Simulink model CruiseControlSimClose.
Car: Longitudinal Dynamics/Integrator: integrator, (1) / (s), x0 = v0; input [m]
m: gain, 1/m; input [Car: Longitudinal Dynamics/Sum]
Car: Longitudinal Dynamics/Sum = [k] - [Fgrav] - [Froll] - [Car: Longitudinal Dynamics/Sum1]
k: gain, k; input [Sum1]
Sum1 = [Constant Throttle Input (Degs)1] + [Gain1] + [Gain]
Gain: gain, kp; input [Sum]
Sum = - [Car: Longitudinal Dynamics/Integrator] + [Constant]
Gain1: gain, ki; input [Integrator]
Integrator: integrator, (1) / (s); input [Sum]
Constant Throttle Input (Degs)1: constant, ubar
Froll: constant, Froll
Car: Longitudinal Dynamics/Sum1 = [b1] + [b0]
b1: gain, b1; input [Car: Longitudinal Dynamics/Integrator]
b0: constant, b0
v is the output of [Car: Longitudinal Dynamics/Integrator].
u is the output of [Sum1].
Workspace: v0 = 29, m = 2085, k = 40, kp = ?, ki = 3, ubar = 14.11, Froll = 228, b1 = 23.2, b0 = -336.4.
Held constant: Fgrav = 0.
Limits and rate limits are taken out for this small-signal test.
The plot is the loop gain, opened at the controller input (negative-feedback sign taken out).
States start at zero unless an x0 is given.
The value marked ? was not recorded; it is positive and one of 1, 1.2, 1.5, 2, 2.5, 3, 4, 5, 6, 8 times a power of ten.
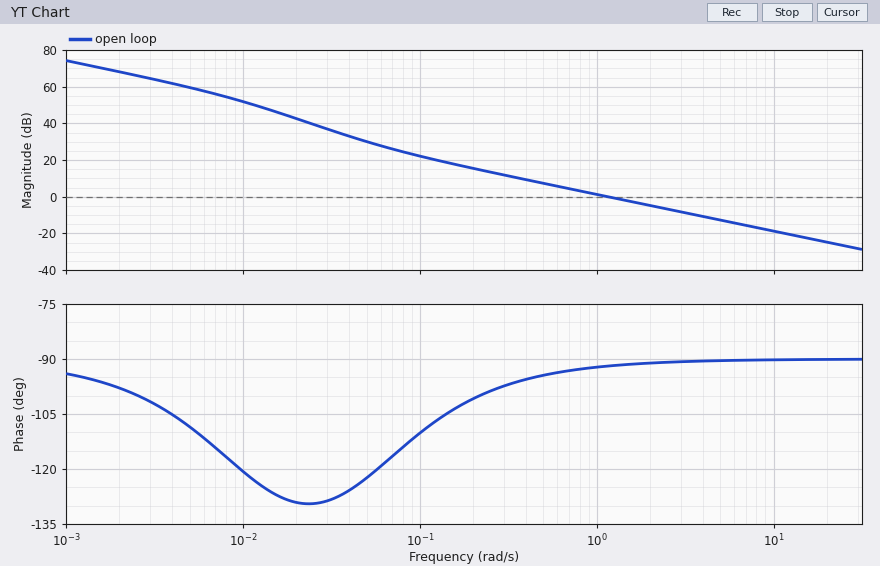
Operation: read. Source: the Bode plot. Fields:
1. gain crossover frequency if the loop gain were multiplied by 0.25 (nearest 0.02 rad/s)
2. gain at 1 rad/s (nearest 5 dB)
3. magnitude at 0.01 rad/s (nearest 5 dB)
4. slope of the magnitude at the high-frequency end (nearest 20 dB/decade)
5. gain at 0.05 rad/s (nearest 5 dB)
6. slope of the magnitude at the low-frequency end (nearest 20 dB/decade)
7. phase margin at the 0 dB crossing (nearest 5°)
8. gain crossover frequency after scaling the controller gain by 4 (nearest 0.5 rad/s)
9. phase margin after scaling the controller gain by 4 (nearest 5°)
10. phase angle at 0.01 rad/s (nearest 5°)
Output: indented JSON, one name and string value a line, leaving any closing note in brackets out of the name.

{
  "gain crossover frequency if the loop gain were multiplied by 0.25": "0.30 rad/s",
  "gain at 1 rad/s": "0 dB",
  "magnitude at 0.01 rad/s": "50 dB",
  "slope of the magnitude at the high-frequency end": "-20 dB/decade",
  "gain at 0.05 rad/s": "30 dB",
  "slope of the magnitude at the low-frequency end": "-20 dB/decade",
  "phase margin at the 0 dB crossing": "90°",
  "gain crossover frequency after scaling the controller gain by 4": "4.5 rad/s",
  "phase margin after scaling the controller gain by 4": "90°",
  "phase angle at 0.01 rad/s": "-120°"
}
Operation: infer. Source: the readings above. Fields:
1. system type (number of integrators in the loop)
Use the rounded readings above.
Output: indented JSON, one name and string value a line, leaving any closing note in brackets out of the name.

{
  "system type": "1"
}
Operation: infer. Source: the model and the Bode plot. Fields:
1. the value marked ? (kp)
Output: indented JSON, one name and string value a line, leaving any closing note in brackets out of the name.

{
  "the value marked ?": "60"
}
